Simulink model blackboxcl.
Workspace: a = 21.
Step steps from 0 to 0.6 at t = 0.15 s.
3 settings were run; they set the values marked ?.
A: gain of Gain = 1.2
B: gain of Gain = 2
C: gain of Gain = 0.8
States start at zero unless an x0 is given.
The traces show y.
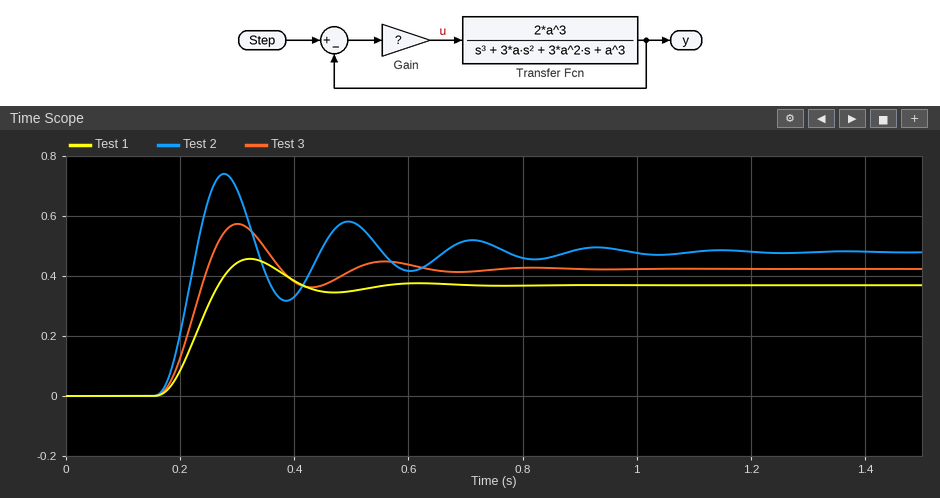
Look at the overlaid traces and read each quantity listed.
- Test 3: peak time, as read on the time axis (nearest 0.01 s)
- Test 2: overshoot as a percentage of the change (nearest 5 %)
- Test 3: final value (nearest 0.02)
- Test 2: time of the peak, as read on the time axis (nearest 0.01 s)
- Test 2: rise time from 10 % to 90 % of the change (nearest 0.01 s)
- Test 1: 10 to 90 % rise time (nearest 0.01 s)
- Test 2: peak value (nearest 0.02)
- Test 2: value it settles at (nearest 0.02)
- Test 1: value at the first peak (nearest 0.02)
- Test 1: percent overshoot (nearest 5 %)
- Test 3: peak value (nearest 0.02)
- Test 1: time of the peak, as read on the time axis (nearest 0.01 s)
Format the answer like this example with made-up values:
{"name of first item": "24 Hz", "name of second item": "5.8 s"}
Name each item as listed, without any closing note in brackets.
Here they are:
{"Test 3: peak time, as read on the time axis": "0.30 s", "Test 2: overshoot as a percentage of the change": "55 %", "Test 3: final value": "0.42", "Test 2: time of the peak, as read on the time axis": "0.28 s", "Test 2: rise time from 10 % to 90 % of the change": "0.05 s", "Test 1: 10 to 90 % rise time": "0.07 s", "Test 2: peak value": "0.74", "Test 2: value it settles at": "0.48", "Test 1: value at the first peak": "0.46", "Test 1: percent overshoot": "25 %", "Test 3: peak value": "0.58", "Test 1: time of the peak, as read on the time axis": "0.32 s"}
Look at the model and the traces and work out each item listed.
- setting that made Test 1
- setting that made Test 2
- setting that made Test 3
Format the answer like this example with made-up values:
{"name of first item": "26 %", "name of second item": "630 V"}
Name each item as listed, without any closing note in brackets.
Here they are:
{"setting that made Test 1": "C", "setting that made Test 2": "B", "setting that made Test 3": "A"}
